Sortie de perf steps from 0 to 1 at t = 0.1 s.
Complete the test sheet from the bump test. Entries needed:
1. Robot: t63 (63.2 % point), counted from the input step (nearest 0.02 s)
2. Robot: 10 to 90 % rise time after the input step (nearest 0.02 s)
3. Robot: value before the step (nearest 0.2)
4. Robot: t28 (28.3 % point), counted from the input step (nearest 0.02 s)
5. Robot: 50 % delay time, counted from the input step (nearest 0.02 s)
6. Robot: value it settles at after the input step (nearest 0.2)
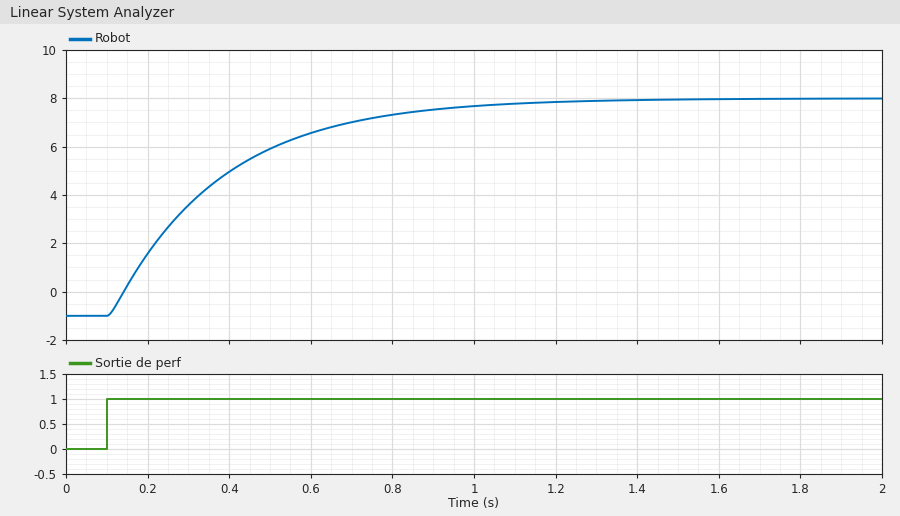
0.28 s
0.58 s
-1.0
0.10 s
0.20 s
8.0
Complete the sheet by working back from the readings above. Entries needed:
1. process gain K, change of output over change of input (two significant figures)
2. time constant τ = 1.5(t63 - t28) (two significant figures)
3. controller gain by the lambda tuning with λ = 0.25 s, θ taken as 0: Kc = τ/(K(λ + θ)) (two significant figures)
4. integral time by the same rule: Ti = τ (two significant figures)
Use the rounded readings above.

9.0
0.27 s
0.12
0.27 s
